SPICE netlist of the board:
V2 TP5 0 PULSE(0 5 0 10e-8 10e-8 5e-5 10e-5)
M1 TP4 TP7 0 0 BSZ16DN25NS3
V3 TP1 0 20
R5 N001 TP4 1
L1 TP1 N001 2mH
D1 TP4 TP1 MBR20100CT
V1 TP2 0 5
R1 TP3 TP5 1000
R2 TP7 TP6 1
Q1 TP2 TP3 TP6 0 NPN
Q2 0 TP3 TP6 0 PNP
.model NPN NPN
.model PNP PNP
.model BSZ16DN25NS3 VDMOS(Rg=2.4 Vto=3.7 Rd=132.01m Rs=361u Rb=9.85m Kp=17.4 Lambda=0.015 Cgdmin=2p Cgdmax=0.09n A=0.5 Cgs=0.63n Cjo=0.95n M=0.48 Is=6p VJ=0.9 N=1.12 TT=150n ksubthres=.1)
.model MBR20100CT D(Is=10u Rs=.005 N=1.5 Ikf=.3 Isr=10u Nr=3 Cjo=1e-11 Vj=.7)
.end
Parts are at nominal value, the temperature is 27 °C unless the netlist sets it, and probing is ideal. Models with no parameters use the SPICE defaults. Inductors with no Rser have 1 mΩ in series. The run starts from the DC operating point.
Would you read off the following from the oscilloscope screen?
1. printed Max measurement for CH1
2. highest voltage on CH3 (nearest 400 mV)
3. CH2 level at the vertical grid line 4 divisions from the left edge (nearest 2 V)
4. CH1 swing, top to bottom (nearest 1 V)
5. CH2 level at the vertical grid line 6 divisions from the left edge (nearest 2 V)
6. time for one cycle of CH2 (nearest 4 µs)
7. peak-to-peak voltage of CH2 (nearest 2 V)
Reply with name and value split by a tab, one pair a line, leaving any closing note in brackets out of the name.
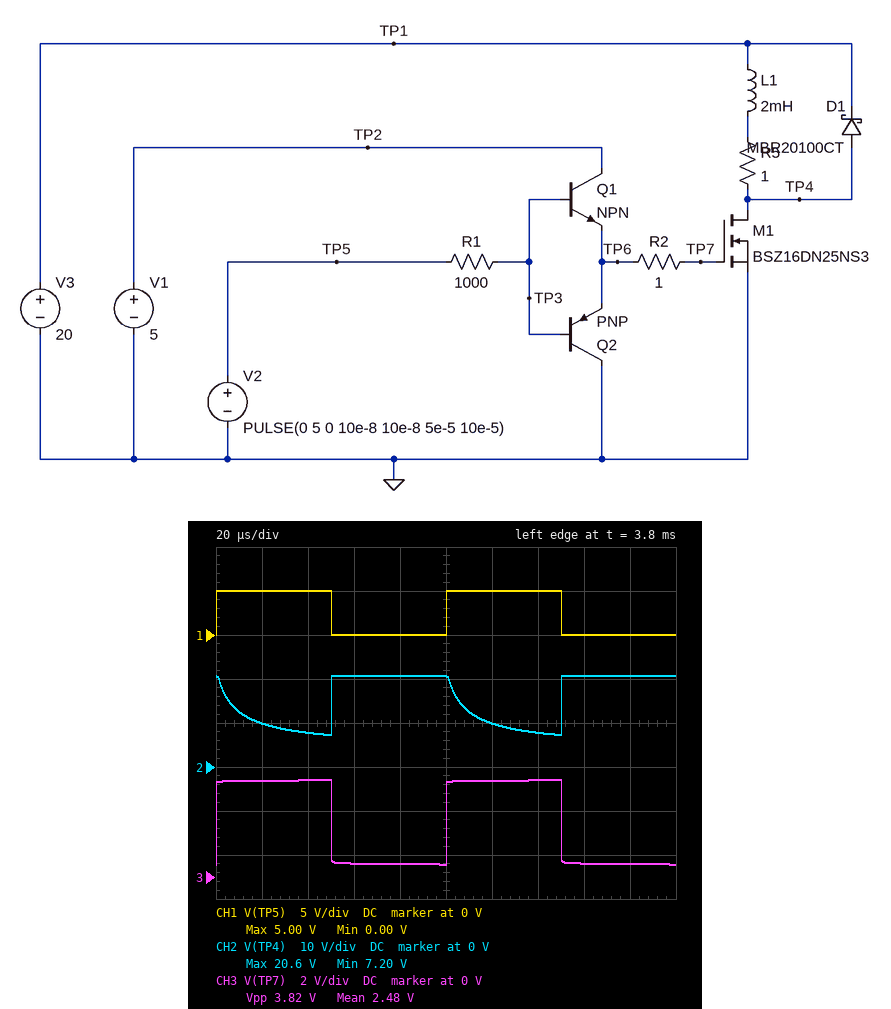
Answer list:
printed Max measurement for CH1	5.00 V
highest voltage on CH3	4.4 V
CH2 level at the vertical grid line 4 divisions from the left edge	20 V
CH1 swing, top to bottom	5 V
CH2 level at the vertical grid line 6 divisions from the left edge	10 V
time for one cycle of CH2	100 µs
peak-to-peak voltage of CH2	14 V
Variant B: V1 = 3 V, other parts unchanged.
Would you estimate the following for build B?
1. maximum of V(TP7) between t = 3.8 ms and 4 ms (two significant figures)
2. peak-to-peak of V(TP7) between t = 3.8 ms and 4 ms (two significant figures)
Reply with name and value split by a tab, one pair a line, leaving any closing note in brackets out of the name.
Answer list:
maximum of V(TP7) between t = 3.8 ms and 4 ms	3.0 V
peak-to-peak of V(TP7) between t = 3.8 ms and 4 ms	2.4 V
